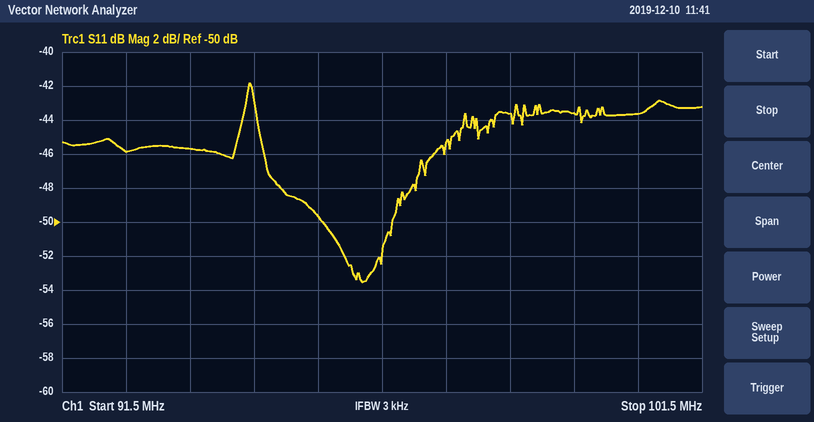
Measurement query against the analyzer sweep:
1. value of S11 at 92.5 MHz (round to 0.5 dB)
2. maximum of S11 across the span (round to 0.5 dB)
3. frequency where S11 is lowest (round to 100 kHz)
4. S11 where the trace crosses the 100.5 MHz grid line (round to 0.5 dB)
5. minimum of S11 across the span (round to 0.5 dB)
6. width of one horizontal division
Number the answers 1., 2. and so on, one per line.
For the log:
1. -46.0 dB
2. -42.0 dB
3. 96.2 MHz
4. -43.5 dB
5. -53.5 dB
6. 1 MHz
